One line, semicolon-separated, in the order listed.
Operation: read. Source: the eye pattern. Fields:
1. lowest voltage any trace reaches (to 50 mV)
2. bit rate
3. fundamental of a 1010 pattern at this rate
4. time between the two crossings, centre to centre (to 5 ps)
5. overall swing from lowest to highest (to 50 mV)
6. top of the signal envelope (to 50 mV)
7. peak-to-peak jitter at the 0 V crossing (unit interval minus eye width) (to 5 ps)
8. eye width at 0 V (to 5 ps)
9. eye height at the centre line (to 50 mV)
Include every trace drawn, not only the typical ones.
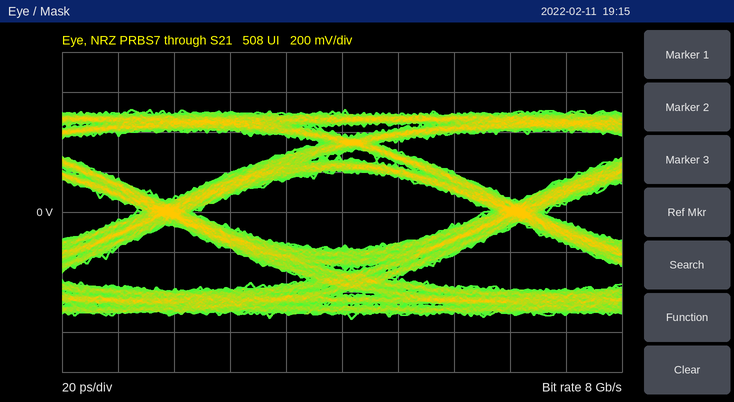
-550 mV; 8 Gb/s; 4 GHz; 125 ps; 1.05 V; 500 mV; 20 ps; 105 ps; 400 mV
